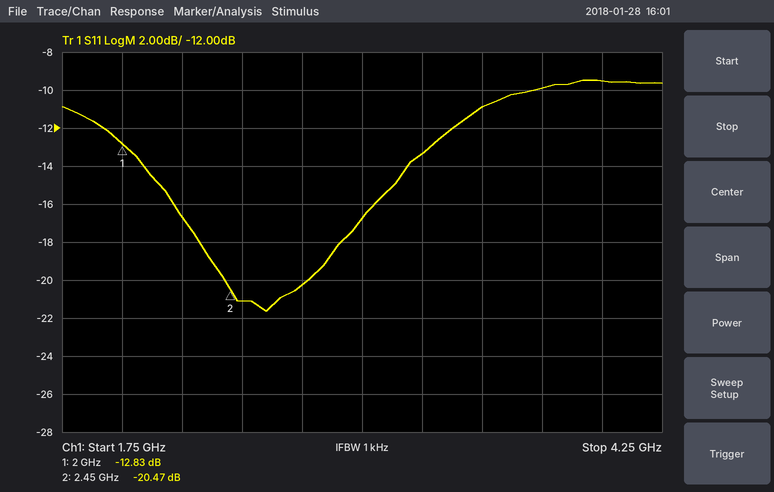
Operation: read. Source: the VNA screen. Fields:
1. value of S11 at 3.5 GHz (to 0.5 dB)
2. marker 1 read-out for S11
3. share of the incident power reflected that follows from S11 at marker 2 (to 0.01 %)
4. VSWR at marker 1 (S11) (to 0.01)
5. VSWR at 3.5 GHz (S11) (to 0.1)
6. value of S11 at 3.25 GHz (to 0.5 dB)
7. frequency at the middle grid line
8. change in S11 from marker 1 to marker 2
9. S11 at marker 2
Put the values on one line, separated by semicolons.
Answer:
-11.0 dB; -12.83 dB; 0.90 %; 1.59; 1.8; -13.5 dB; 3 GHz; -7.64 dB; -20.47 dB
